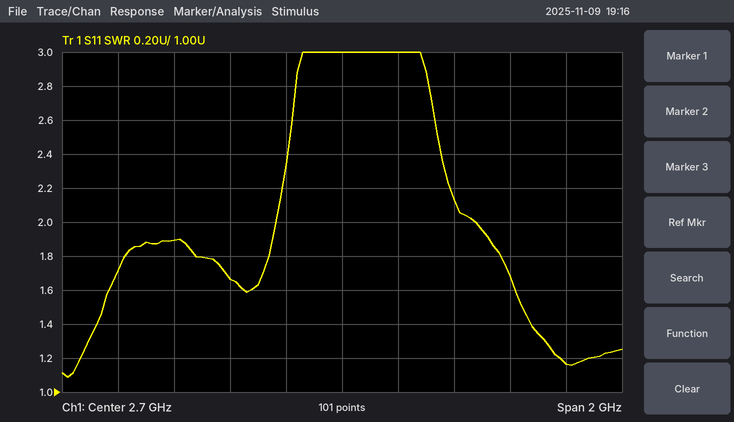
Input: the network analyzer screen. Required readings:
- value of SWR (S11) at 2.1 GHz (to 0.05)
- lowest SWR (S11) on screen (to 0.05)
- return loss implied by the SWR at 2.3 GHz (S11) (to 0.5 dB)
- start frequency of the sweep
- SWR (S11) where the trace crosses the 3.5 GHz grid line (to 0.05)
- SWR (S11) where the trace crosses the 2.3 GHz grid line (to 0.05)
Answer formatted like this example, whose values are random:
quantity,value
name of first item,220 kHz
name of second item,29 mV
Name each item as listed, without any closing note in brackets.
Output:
quantity,value
value of SWR (S11) at 2.1 GHz,1.90
lowest SWR (S11) on screen,1.10
return loss implied by the SWR at 2.3 GHz (S11),12.0 dB
start frequency of the sweep,1.7 GHz
SWR (S11) where the trace crosses the 3.5 GHz grid line,1.15
SWR (S11) where the trace crosses the 2.3 GHz grid line,1.65
